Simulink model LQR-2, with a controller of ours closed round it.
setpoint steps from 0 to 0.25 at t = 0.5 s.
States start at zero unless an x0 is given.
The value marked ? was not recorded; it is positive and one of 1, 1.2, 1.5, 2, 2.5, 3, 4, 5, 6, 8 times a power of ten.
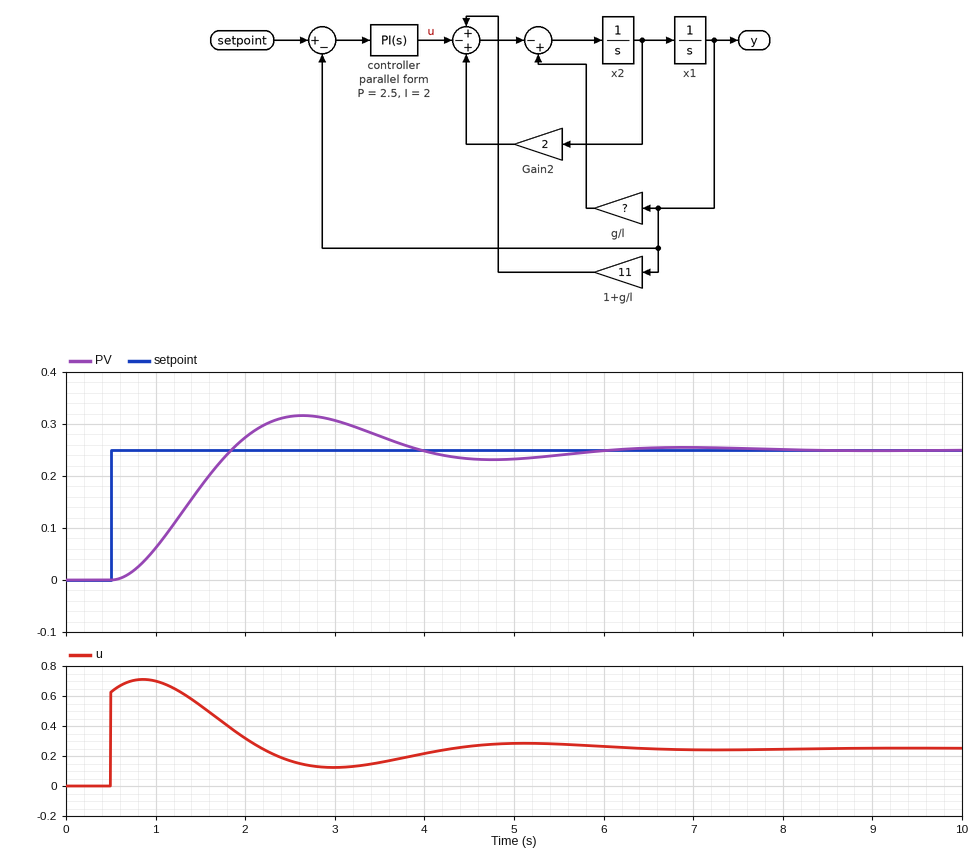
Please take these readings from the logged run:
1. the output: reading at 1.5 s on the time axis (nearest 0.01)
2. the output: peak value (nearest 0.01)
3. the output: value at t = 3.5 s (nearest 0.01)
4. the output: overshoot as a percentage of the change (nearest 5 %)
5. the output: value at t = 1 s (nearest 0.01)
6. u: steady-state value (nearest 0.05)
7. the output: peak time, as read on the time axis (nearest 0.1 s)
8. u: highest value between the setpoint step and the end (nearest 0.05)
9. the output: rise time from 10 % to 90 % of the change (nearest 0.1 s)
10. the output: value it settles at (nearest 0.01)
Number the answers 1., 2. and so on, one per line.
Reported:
1. 0.18
2. 0.32
3. 0.28
4. 25 %
5. 0.06
6. 0.25
7. 2.6 s
8. 0.70
9. 0.9 s
10. 0.25
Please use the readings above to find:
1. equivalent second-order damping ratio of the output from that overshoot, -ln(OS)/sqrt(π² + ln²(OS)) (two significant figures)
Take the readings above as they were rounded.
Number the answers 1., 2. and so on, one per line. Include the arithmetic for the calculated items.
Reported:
1. ln(0.25) = -1.386; 1.386 / sqrt(9.870 + 1.922) = 0.40
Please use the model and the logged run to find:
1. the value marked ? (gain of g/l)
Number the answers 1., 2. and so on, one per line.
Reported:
1. 10
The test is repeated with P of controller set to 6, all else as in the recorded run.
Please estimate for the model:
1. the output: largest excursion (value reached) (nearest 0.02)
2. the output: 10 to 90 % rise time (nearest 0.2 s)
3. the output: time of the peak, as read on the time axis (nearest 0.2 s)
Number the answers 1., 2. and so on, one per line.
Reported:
1. 0.32
2. 0.6 s
3. 1.8 s
